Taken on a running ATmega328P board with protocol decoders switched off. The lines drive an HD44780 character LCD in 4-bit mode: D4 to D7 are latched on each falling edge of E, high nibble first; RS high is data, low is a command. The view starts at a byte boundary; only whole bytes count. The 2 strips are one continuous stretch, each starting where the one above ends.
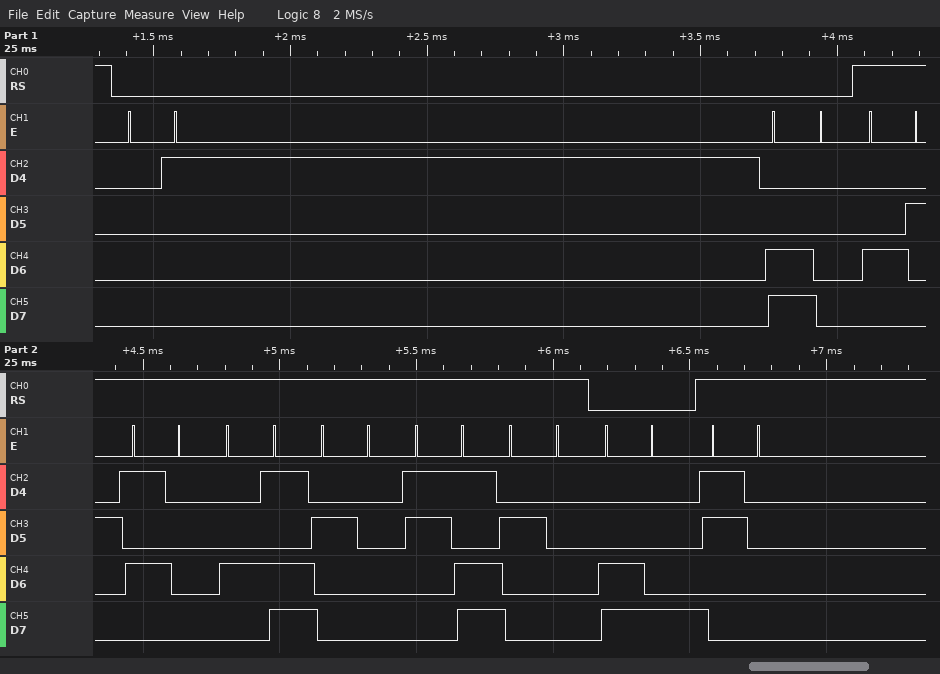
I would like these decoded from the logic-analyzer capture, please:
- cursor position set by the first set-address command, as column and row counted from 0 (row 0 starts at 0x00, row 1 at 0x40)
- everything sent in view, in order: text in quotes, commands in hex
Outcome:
column 0, row 1
0x01 0xC0 "BPM = " 0xC8 "0"
